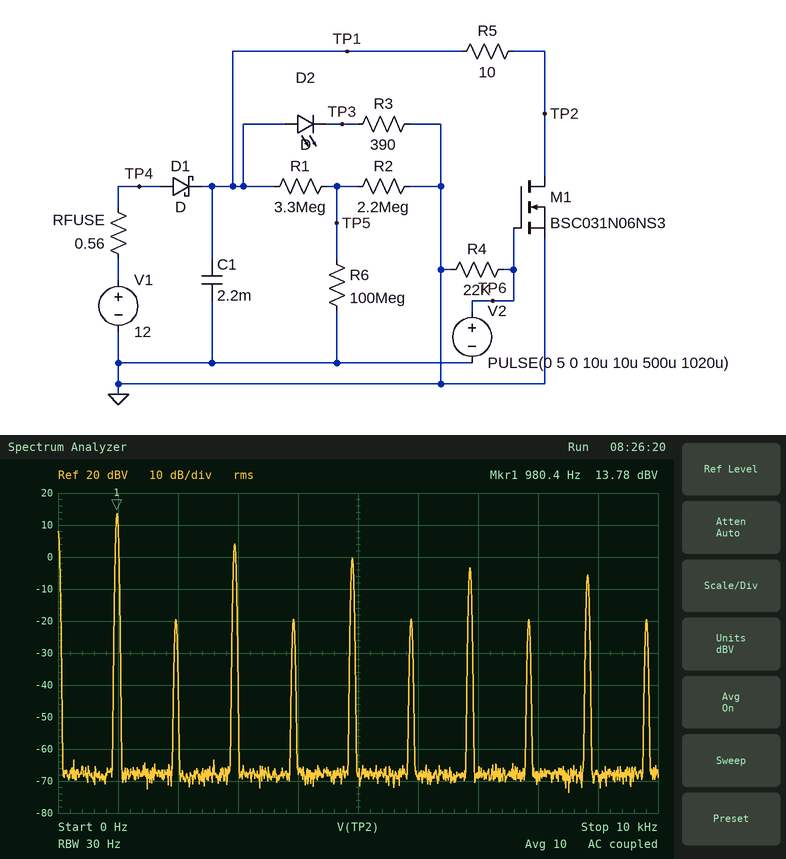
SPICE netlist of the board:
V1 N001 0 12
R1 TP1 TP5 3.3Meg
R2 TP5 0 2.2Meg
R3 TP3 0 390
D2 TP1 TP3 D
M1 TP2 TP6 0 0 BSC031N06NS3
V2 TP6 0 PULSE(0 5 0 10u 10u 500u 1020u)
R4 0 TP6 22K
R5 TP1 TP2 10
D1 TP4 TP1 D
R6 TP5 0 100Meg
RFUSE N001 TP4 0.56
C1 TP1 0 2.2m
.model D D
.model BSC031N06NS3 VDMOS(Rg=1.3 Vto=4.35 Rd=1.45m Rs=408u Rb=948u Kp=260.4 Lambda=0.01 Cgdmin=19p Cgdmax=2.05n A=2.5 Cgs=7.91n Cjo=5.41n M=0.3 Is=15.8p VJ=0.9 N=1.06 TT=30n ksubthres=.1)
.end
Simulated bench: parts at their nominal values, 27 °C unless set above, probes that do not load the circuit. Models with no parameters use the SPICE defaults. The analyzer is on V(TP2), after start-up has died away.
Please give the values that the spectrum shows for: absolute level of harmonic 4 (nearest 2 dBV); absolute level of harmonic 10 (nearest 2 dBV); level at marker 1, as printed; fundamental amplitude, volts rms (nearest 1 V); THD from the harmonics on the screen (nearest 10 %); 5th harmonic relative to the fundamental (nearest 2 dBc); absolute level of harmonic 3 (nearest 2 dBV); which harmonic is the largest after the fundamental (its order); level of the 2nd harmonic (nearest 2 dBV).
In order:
-20 dBV
-20 dBV
13.78 dBV
5 V
40 %
-14 dBc
4 dBV
3
-20 dBV
